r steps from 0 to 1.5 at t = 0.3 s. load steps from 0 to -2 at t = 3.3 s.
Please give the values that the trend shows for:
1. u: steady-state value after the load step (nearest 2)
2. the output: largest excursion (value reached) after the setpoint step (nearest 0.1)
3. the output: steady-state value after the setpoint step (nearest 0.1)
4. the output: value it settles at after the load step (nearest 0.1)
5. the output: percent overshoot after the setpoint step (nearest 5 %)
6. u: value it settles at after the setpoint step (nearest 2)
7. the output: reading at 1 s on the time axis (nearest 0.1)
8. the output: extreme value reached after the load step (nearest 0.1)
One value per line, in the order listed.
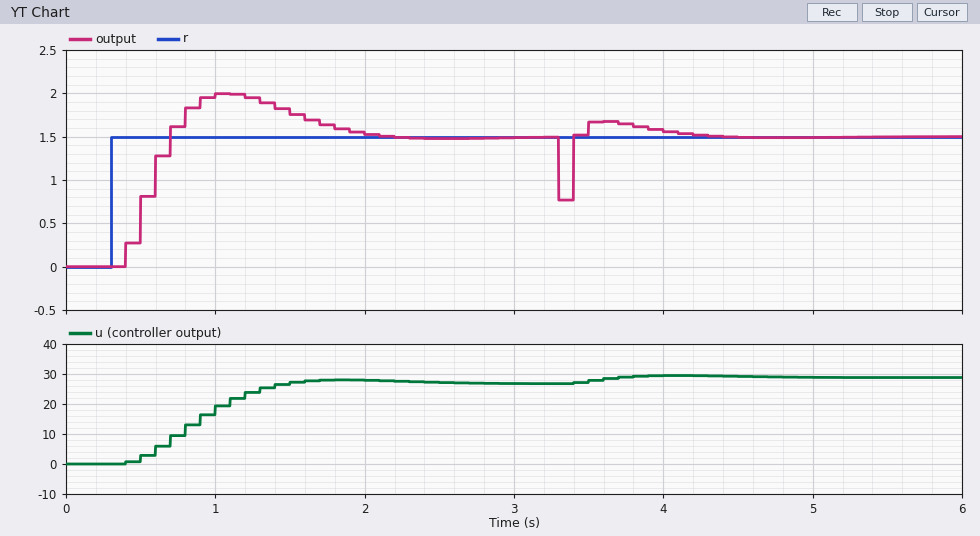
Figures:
28
2.0
1.5
1.5
35 %
26
2.0
0.8
